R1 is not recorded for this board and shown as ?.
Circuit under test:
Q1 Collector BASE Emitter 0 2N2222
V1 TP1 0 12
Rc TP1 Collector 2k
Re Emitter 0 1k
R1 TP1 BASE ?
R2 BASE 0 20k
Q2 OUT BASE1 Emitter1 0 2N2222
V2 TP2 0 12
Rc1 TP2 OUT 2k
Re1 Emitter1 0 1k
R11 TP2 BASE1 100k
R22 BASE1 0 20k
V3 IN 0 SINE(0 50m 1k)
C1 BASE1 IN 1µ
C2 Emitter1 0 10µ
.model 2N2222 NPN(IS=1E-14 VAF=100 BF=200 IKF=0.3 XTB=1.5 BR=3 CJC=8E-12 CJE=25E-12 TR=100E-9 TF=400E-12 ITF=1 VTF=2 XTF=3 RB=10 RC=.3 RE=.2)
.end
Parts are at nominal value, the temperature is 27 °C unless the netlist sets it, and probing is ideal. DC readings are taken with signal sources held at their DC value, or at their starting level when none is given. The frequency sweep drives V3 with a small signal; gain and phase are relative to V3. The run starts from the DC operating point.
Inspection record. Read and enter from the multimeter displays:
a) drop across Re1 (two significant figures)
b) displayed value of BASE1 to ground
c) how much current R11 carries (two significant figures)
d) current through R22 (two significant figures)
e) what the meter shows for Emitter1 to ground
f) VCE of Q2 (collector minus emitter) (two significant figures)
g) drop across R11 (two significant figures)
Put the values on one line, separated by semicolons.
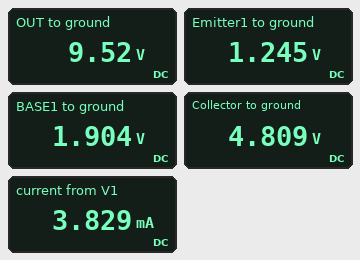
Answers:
1.2 V; 1.904 V; 100 µA; 95 µA; 1.245 V; 8.3 V; 10 V
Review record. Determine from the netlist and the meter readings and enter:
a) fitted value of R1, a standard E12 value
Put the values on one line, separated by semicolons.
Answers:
33 kΩ
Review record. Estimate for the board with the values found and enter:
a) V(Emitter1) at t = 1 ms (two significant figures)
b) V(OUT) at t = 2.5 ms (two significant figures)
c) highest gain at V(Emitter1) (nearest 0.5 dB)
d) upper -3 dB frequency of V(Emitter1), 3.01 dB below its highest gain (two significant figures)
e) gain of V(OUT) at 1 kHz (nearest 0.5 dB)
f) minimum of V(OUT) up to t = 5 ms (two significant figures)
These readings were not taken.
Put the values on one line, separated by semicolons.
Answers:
1.2 V; 11 V; -0.5 dB; 810 Hz; 37.0 dB; 5.4 V
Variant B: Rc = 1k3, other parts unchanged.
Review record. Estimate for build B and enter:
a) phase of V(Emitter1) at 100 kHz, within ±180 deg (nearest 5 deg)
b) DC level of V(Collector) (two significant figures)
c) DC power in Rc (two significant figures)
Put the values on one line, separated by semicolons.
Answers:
-90 deg; 7.3 V; 17 mW
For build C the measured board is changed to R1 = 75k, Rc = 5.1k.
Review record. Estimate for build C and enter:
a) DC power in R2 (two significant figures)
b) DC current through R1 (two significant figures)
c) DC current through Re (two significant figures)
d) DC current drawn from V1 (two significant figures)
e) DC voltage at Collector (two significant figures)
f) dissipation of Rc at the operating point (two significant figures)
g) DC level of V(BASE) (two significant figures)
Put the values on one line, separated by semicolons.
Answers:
290 µW; 130 µA; 1.7 mA; 1.8 mA; 3.3 V; 15 mW; 2.4 V
